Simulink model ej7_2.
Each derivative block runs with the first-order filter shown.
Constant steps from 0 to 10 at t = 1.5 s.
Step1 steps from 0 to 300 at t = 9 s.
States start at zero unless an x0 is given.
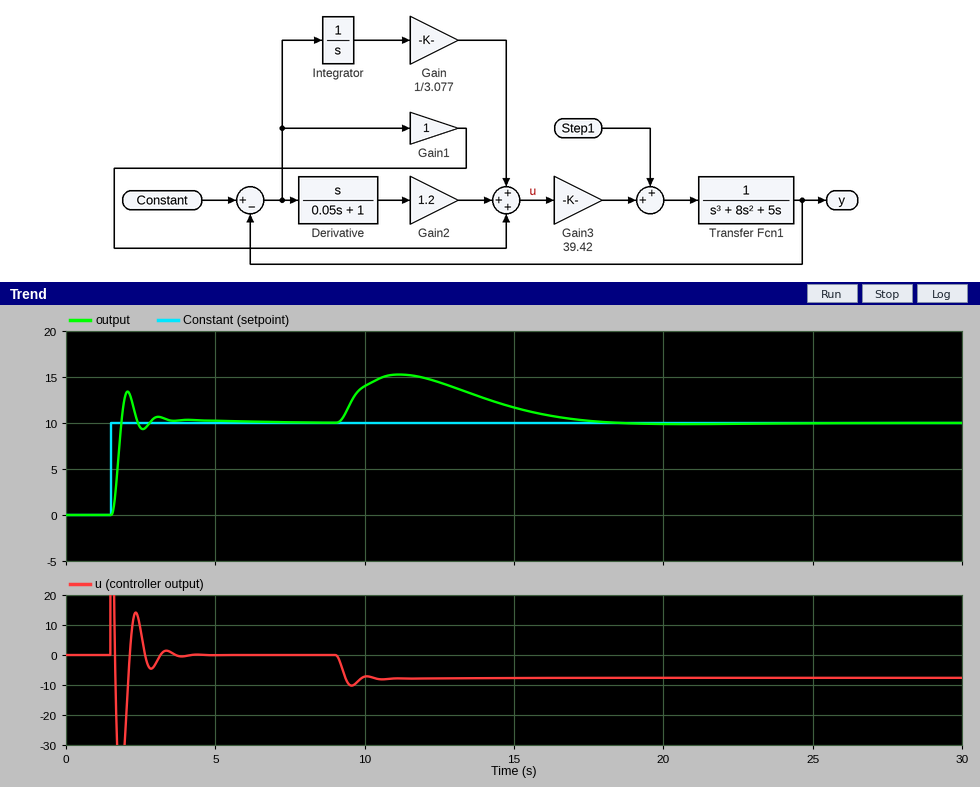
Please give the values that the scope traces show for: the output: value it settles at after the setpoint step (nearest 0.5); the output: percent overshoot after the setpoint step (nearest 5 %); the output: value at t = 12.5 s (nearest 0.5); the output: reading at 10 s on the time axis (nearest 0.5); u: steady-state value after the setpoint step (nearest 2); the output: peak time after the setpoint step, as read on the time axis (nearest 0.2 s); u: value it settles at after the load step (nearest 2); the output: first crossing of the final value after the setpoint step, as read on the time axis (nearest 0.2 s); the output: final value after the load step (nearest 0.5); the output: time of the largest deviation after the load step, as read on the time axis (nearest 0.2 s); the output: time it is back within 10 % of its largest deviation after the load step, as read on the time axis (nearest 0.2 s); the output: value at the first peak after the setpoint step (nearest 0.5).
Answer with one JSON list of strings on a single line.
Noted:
["10.0", "35 %", "14.5", "14.0", "0", "2.0 s", "-8", "1.8 s", "10.0", "11.2 s", "16.8 s", "13.5"]
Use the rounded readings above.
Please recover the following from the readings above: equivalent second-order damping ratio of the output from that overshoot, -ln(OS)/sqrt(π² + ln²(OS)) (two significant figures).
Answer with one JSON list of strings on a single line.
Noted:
["0.32"]
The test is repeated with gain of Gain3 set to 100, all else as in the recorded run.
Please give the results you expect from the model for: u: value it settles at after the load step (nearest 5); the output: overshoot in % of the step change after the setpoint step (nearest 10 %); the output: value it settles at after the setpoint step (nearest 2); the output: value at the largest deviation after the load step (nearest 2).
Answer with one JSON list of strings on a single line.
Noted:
["-5", "70 %", "10", "12"]
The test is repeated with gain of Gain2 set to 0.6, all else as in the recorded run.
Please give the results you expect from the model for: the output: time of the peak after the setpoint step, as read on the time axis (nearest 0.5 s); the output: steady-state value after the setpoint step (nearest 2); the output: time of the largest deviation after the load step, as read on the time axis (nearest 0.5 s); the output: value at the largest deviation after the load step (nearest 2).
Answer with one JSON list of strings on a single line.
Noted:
["2.5 s", "10", "10.5 s", "16"]
